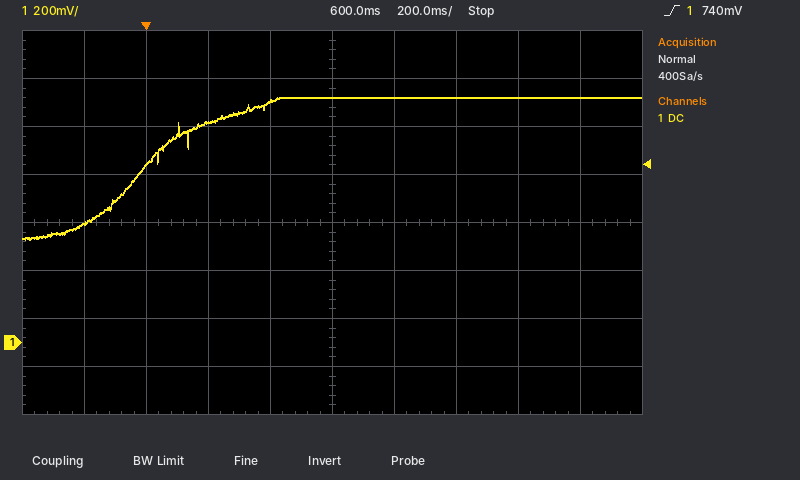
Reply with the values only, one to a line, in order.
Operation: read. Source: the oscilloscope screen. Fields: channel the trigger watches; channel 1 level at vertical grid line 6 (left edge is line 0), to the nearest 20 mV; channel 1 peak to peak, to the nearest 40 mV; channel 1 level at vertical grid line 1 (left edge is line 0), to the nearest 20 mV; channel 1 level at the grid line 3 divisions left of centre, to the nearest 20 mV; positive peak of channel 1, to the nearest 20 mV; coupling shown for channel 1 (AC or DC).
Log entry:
channel 1
1.02 V
600 mV
500 mV
740 mV
1.02 V
DC
